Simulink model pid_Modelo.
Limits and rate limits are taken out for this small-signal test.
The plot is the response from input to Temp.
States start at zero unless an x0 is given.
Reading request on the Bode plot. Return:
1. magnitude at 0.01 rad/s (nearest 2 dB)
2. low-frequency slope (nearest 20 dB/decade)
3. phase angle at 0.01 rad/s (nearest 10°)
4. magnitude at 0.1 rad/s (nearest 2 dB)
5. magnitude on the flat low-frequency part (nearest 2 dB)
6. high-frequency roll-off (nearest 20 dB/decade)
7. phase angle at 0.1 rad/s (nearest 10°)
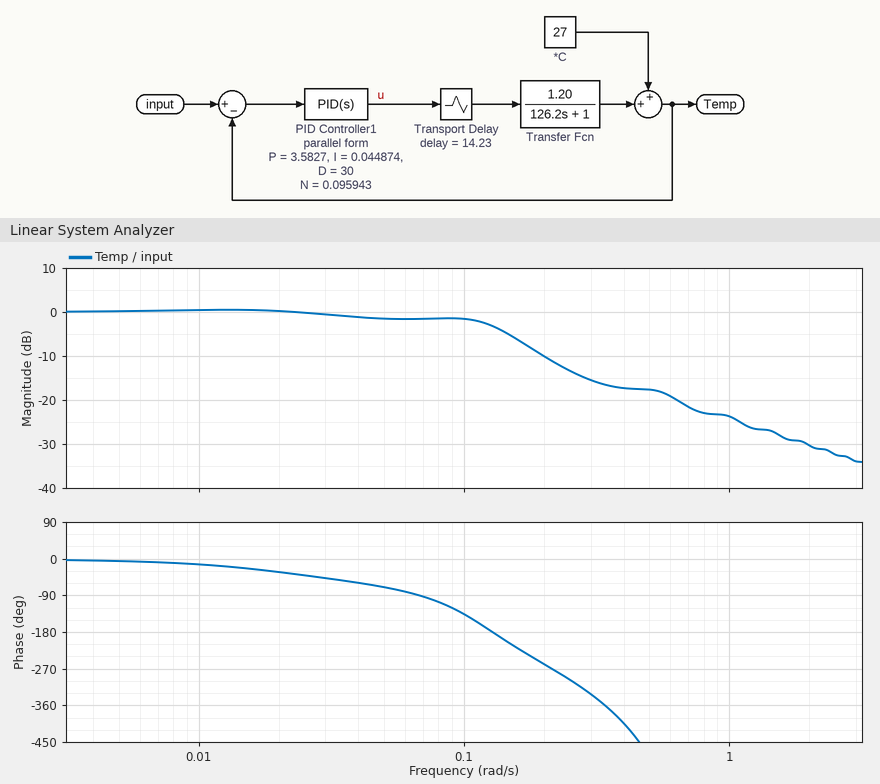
0 dB
0 dB/decade
-10°
-2 dB
0 dB
-20 dB/decade
-140°
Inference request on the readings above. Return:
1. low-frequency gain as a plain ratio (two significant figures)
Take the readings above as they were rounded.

1.0
